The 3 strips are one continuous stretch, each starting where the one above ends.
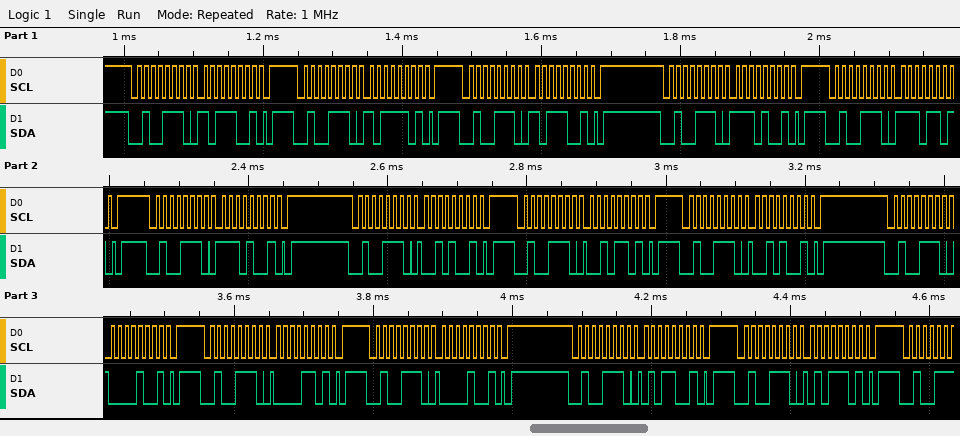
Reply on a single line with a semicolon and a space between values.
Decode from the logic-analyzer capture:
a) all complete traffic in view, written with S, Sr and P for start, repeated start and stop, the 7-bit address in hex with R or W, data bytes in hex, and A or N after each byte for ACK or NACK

S 27W A B9 A P S 27W A BD A P S 27W A B9 A P S 27W A E9 A P S 27W A ED A P S 27W A E9 A P S 27W A 29 A P S 27W A 2D A P S 27W A 29 A P S 27W A 09 A P S 27W A 0D A P S 27W A 09 A P S 27W A 59 A P S 27W A 5D A P
